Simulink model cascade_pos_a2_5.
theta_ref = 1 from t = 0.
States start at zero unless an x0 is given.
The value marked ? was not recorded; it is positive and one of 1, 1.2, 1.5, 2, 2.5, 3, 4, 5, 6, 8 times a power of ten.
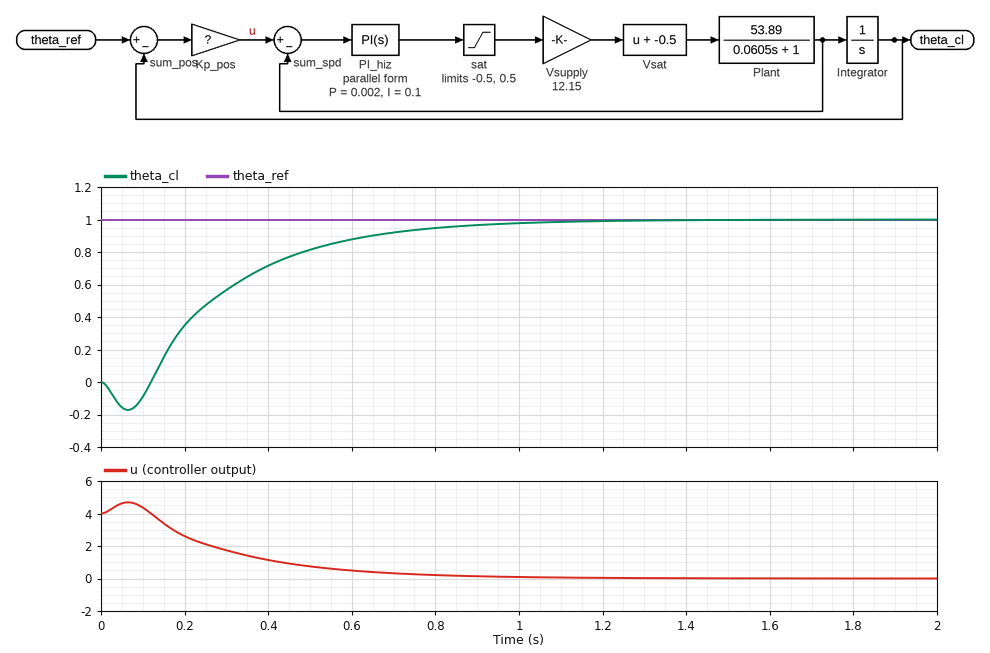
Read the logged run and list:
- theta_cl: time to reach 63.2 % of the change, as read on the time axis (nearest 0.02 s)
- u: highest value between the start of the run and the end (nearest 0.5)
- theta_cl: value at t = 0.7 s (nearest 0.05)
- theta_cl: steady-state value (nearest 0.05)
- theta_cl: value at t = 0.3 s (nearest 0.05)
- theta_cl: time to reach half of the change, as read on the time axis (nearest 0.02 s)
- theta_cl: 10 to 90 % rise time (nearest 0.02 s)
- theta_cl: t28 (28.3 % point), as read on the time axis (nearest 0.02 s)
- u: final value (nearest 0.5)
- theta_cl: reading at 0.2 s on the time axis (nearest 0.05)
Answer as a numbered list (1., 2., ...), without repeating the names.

1. 0.34 s
2. 4.5
3. 0.90
4. 1.00
5. 0.55
6. 0.26 s
7. 0.50 s
8. 0.18 s
9. 0.0
10. 0.35
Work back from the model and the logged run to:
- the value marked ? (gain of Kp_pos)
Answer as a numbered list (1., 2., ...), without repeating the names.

1. 4
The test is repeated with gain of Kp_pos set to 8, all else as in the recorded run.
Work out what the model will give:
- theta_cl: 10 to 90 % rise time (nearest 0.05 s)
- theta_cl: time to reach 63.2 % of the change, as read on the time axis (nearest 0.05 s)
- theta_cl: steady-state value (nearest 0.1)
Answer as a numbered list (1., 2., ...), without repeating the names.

1. 0.25 s
2. 0.15 s
3. 1.0
